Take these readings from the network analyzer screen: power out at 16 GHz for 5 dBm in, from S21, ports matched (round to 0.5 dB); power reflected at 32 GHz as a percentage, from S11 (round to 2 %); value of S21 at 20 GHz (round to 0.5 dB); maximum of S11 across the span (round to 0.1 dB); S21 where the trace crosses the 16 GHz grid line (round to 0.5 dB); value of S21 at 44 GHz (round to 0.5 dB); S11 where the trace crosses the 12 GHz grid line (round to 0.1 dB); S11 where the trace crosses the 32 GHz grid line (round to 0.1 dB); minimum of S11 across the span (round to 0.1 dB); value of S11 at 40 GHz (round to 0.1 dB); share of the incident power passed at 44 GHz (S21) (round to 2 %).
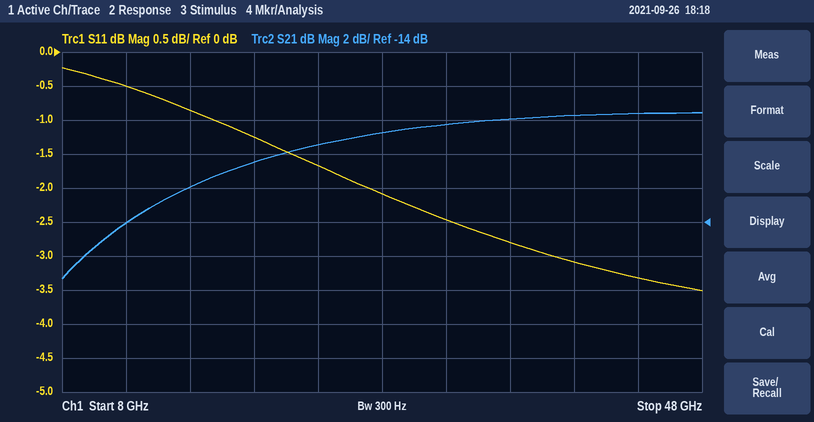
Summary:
-7.0 dBm
56 %
-10.5 dB
-0.2 dB
-12.0 dB
-7.5 dB
-0.5 dB
-2.5 dB
-3.5 dB
-3.1 dB
18 %
